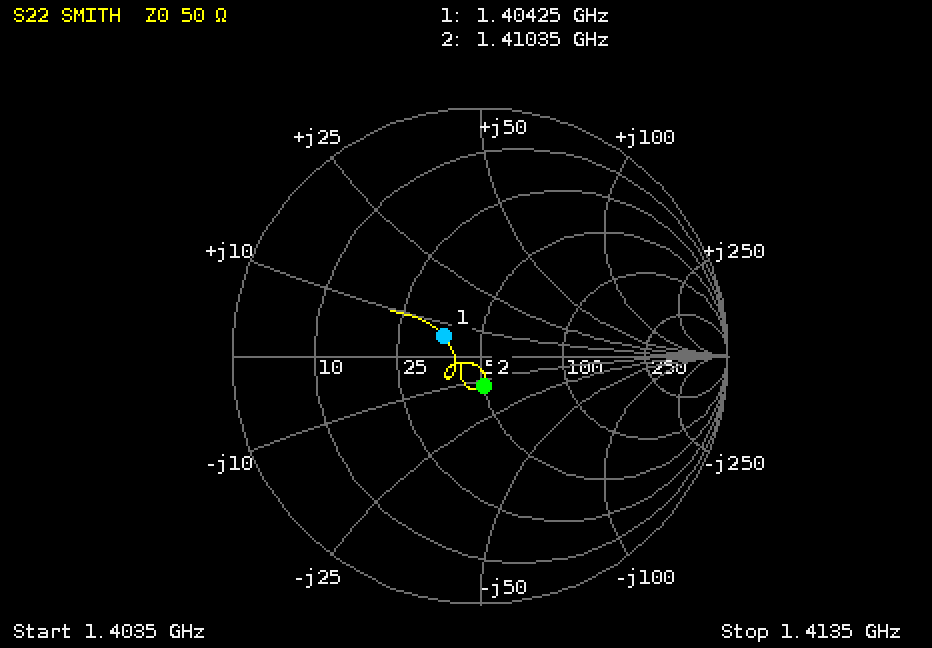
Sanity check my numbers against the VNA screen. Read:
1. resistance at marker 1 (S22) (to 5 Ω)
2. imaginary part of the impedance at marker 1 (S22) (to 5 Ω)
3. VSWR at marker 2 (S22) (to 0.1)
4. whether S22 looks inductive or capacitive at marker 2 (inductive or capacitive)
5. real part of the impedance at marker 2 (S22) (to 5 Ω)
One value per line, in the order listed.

35 Ω
+5 Ω
1.3
capacitive
50 Ω
